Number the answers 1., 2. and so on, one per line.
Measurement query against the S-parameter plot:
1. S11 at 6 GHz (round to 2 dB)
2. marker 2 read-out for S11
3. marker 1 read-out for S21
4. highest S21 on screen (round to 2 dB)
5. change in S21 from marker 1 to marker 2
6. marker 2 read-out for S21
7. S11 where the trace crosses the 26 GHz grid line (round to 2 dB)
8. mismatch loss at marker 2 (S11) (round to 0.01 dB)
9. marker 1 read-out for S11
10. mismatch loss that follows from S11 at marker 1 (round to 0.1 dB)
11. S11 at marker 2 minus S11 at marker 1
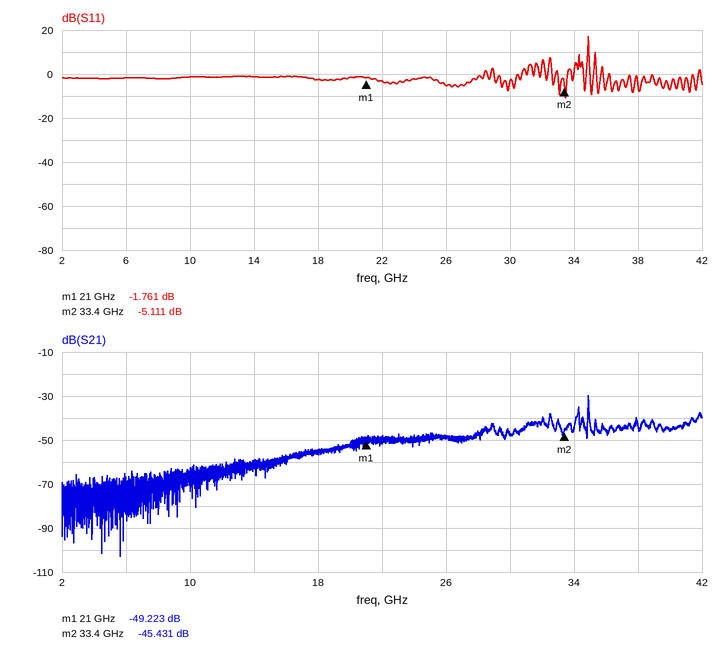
1. -2 dB
2. -5.111 dB
3. -49.223 dB
4. -30 dB
5. 3.792 dB
6. -45.431 dB
7. -6 dB
8. 1.60 dB
9. -1.761 dB
10. 4.8 dB
11. -3.350 dB
